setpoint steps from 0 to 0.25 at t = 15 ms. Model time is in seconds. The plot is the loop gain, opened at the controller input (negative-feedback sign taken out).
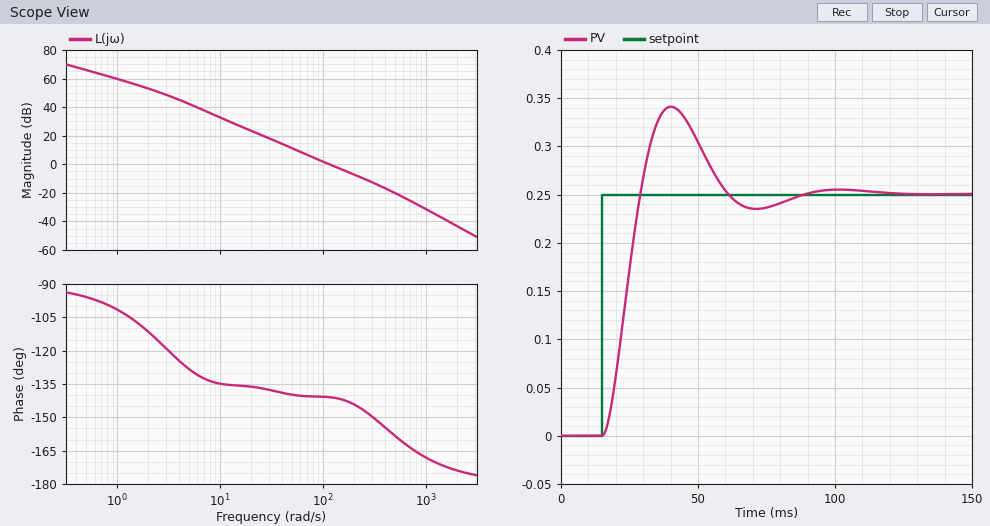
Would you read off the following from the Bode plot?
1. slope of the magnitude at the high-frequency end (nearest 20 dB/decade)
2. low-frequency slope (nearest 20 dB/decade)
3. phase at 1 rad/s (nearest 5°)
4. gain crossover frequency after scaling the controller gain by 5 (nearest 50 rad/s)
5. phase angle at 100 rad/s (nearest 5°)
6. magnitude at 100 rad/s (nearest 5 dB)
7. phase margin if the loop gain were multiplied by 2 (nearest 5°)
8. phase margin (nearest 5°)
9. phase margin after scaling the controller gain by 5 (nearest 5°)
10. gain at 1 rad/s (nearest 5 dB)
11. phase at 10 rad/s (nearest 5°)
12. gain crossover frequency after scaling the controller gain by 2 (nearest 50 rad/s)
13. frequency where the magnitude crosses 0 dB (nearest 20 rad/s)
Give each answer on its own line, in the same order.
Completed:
-40 dB/decade
-20 dB/decade
-100°
350 rad/s
-140°
0 dB
35°
40°
30°
60 dB
-135°
200 rad/s
120 rad/s
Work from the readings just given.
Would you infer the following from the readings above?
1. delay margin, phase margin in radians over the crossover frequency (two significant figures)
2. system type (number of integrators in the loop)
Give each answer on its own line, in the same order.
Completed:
0.0058 s
1
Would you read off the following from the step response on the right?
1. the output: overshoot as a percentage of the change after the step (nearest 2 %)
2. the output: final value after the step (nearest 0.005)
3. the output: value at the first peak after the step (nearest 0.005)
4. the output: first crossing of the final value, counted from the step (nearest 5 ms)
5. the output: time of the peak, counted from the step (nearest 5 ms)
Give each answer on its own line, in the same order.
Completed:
36 %
0.250
0.340
15 ms
25 ms
